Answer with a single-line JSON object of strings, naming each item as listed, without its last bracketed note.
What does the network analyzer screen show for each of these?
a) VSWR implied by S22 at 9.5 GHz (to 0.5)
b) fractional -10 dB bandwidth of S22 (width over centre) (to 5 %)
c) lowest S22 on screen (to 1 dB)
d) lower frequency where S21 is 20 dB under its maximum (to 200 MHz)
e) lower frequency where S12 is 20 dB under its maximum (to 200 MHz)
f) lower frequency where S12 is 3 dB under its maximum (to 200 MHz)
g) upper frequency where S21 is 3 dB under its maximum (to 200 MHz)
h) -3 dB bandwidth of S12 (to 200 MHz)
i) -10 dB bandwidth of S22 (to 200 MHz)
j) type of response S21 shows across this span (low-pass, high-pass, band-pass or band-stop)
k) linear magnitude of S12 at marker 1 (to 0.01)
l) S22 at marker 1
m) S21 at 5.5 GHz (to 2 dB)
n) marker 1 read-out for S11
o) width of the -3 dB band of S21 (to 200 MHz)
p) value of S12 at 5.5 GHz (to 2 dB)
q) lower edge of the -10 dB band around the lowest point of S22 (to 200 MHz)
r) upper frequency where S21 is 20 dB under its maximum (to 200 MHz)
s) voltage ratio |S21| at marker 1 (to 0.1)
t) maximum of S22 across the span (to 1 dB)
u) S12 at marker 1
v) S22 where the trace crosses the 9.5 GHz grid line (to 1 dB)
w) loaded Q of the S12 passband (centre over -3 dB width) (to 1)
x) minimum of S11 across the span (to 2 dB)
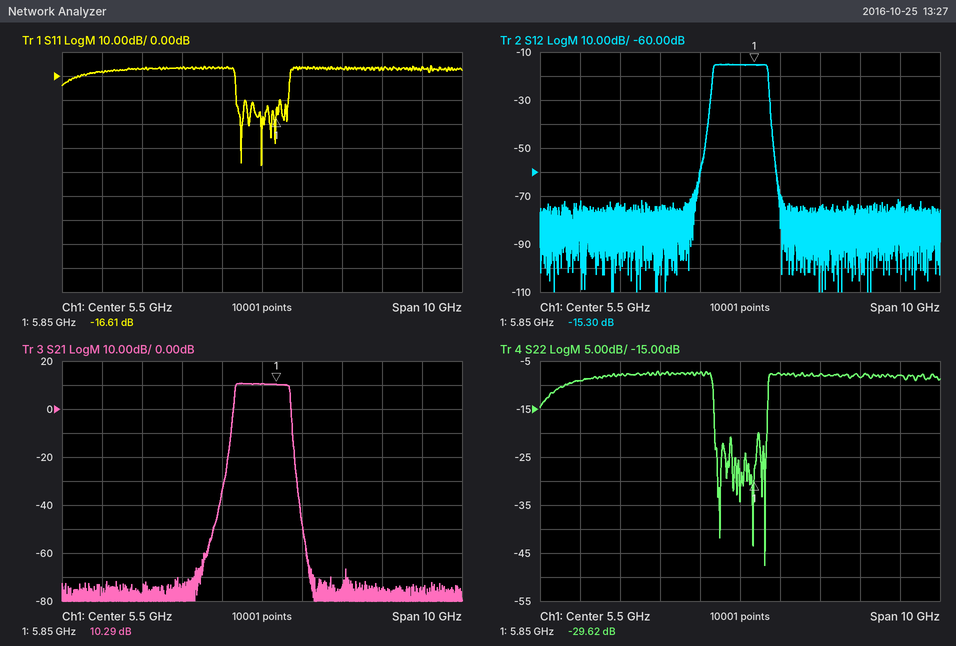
{"VSWR implied by S22 at 9.5 GHz": "2.5", "fractional -10 dB bandwidth of S22 (width over centre)": "25 %", "lowest S22 on screen": "-48 dB", "lower frequency where S21 is 20 dB under its maximum": "4.8 GHz", "lower frequency where S12 is 20 dB under its maximum": "4.8 GHz", "lower frequency where S12 is 3 dB under its maximum": "4.8 GHz", "upper frequency where S21 is 3 dB under its maximum": "6.2 GHz", "-3 dB bandwidth of S12": "1.4 GHz", "-10 dB bandwidth of S22": "1.4 GHz", "type of response S21 shows across this span": "band-pass", "linear magnitude of S12 at marker 1": "0.17", "S22 at marker 1": "-29.62 dB", "S21 at 5.5 GHz": "10 dB", "marker 1 read-out for S11": "-16.61 dB", "width of the -3 dB band of S21": "1.4 GHz", "value of S12 at 5.5 GHz": "-16 dB", "lower edge of the -10 dB band around the lowest point of S22": "4.8 GHz", "upper frequency where S21 is 20 dB under its maximum": "6.2 GHz", "voltage ratio |S21| at marker 1": "3.3", "maximum of S22 across the span": "-7 dB", "S12 at marker 1": "-15.30 dB", "S22 where the trace crosses the 9.5 GHz grid line": "-8 dB", "loaded Q of the S12 passband (centre over -3 dB width)": "4", "minimum of S11 across the span": "-38 dB"}
